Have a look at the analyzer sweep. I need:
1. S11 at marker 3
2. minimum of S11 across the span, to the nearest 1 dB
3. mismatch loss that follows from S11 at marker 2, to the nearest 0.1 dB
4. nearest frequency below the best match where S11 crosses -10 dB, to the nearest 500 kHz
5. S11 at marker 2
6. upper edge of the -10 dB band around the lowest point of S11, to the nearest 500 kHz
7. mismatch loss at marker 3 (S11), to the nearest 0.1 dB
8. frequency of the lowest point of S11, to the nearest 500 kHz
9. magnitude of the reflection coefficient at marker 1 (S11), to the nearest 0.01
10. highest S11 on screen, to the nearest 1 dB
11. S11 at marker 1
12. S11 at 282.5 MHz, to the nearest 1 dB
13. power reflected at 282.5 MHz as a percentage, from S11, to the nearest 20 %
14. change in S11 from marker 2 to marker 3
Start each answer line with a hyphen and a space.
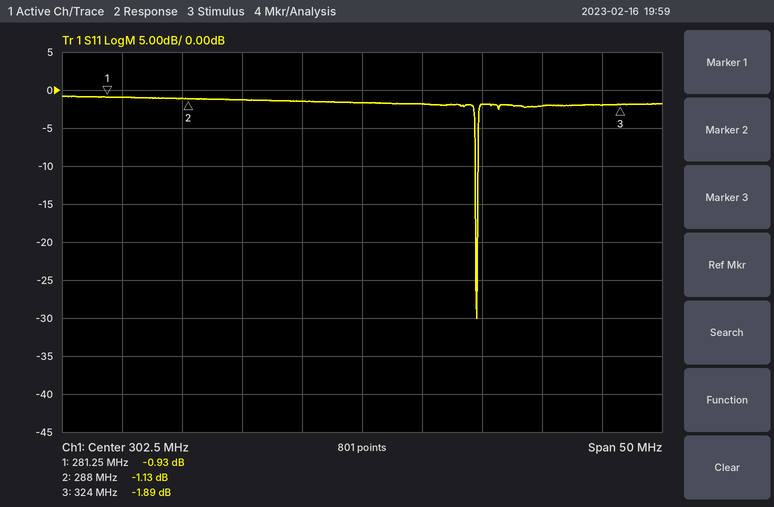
- -1.89 dB
- -30 dB
- 6.4 dB
- 312.0 MHz
- -1.13 dB
- 312.0 MHz
- 4.5 dB
- 312.0 MHz
- 0.90
- -1 dB
- -0.93 dB
- -1 dB
- 80 %
- -0.76 dB
